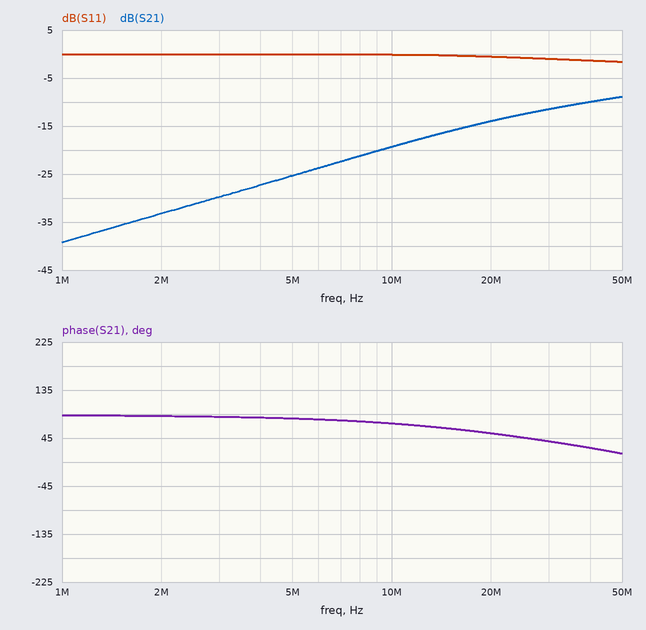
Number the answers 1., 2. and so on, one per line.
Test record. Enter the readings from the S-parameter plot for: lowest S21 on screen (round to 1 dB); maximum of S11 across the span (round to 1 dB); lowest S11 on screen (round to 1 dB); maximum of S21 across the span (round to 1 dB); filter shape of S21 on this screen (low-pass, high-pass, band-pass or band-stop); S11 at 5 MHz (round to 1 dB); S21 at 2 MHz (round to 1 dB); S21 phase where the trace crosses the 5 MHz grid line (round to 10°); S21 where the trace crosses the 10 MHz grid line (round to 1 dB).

1. -39 dB
2. 0 dB
3. -2 dB
4. -9 dB
5. high-pass
6. 0 dB
7. -33 dB
8. 80°
9. -19 dB
